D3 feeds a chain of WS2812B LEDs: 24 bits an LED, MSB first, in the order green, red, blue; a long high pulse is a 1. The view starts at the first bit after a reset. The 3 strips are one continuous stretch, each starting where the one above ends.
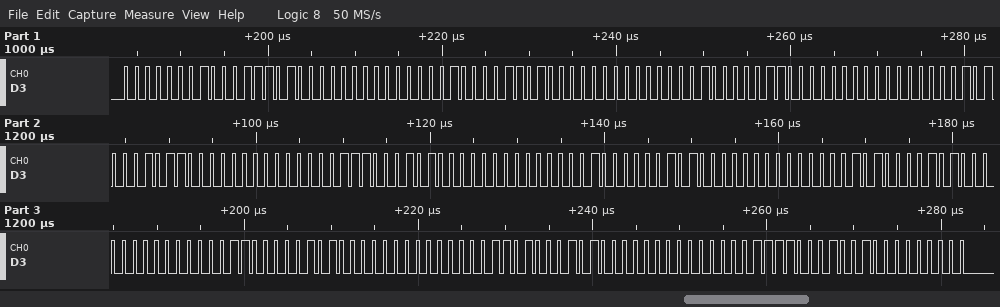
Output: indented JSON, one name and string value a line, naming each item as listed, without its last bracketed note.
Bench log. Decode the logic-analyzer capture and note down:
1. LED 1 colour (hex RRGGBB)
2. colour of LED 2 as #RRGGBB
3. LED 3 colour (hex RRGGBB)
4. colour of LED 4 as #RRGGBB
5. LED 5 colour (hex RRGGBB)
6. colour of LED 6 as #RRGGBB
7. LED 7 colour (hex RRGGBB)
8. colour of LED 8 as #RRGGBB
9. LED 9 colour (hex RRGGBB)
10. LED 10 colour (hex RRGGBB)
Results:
{
  "LED 1 colour": "#1D0100",
  "colour of LED 2 as #RRGGBB": "#1A0200",
  "LED 3 colour": "#180400",
  "colour of LED 4 as #RRGGBB": "#160500",
  "LED 5 colour": "#140700",
  "colour of LED 6 as #RRGGBB": "#140800",
  "LED 7 colour": "#140A00",
  "colour of LED 8 as #RRGGBB": "#140C00",
  "LED 9 colour": "#140D00",
  "LED 10 colour": "#120F00"
}
